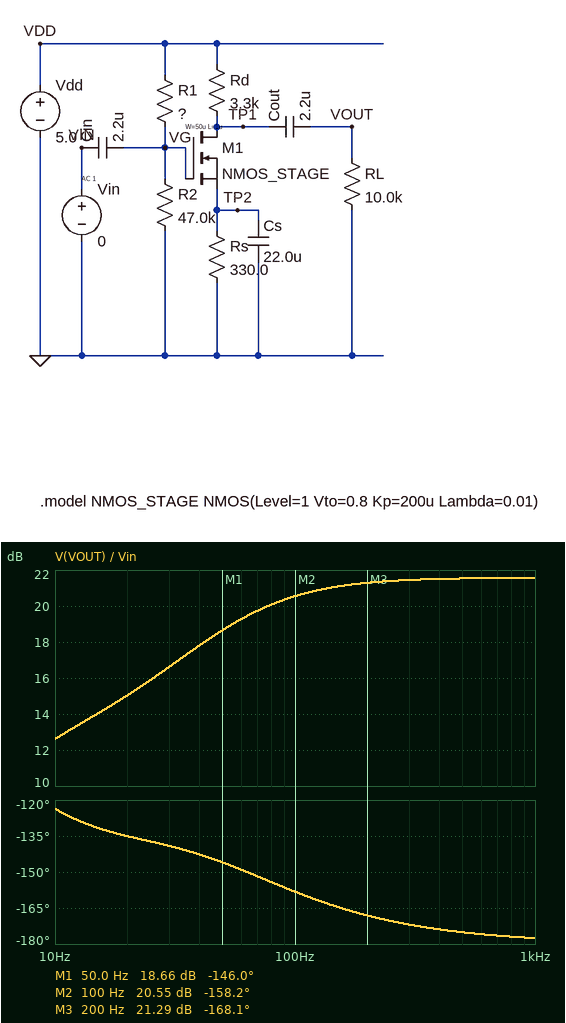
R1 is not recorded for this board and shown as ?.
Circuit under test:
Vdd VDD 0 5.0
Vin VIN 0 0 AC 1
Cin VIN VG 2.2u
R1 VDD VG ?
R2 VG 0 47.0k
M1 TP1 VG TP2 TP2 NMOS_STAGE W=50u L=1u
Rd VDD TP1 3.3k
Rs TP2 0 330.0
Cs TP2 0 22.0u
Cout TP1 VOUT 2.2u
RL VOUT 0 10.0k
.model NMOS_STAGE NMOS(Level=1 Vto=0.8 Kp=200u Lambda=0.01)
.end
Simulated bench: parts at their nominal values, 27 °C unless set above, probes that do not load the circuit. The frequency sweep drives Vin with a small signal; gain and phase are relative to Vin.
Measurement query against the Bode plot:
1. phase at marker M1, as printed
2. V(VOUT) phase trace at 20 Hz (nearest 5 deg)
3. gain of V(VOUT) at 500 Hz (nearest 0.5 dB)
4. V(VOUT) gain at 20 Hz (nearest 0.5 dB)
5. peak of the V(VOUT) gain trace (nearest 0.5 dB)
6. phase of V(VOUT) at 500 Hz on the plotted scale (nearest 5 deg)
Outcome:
-146.0 deg
-135 deg
21.5 dB
15.0 dB
21.5 dB
-175 deg
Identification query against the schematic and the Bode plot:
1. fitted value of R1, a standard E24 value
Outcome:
91 kΩ
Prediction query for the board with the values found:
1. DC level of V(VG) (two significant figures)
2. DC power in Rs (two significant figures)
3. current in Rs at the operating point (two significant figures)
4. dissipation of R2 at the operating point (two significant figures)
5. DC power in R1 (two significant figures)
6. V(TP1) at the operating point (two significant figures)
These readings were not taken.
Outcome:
1.7 V
500 µW
1.2 mA
62 µW
120 µW
930 mV
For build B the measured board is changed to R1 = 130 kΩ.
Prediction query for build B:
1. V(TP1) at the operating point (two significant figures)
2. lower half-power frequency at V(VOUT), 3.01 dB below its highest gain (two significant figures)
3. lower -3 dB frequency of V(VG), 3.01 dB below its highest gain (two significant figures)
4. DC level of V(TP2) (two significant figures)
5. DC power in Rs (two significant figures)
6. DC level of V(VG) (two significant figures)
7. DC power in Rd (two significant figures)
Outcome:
3.1 V
36 Hz
2.1 Hz
190 mV
110 µW
1.3 V
1.1 mW
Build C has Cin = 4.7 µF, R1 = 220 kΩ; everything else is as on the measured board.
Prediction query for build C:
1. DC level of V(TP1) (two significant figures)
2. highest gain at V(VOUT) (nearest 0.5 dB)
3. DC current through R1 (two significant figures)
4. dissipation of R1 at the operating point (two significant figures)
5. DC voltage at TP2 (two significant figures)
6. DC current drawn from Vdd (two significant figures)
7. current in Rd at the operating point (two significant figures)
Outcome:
4.9 V
5.5 dB
19 µA
77 µW
8.8 mV
45 µA
27 µA
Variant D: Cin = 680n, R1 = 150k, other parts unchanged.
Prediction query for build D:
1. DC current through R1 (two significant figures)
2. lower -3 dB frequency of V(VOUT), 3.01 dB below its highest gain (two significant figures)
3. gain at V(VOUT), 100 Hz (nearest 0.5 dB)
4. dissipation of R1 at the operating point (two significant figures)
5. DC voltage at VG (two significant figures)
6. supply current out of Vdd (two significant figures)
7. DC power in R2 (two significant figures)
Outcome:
25 µA
32 Hz
16.0 dB
97 µW
1.2 V
400 µA
30 µW
